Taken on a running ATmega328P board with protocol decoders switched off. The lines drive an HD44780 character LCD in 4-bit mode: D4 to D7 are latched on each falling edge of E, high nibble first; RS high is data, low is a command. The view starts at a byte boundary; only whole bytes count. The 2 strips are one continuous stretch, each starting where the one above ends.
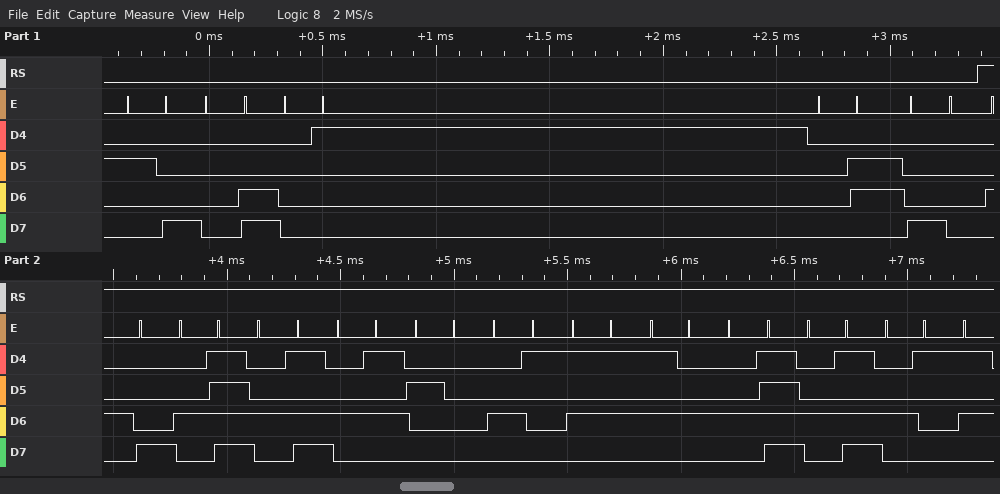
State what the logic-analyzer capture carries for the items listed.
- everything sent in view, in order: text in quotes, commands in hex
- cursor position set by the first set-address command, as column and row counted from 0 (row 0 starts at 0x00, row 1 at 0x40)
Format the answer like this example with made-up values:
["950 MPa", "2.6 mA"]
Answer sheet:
["0x28 0x0C 0x01 0x06 0x80 \"HOME AUTOMA\"", "column 0, row 0"]
